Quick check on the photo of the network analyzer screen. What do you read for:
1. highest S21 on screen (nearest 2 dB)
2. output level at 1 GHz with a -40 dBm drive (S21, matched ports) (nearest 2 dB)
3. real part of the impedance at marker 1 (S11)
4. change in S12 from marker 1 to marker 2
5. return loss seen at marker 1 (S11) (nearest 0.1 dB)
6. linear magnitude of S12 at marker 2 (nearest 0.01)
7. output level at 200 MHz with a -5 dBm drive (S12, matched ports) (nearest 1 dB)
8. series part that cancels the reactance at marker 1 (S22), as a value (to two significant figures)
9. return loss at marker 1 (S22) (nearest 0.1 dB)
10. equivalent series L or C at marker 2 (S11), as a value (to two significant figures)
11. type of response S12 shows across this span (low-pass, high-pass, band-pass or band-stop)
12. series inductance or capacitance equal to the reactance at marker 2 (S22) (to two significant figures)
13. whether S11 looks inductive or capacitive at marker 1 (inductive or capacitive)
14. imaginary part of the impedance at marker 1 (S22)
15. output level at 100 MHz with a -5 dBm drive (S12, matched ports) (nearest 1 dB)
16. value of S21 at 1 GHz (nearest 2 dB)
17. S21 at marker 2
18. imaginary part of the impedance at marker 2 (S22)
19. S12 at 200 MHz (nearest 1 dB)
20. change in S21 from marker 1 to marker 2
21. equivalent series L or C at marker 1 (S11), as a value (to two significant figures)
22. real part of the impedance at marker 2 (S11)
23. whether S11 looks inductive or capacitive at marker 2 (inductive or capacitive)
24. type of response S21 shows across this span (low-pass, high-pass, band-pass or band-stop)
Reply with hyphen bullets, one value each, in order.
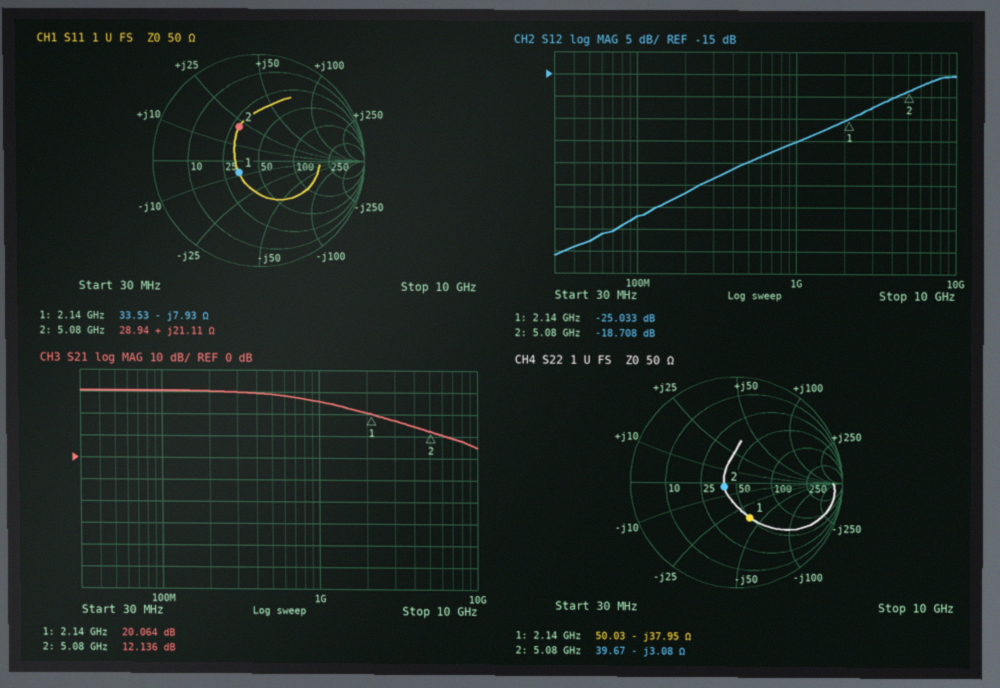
- 30 dB
- -14 dBm
- 33.53 Ω
- 6.325 dB
- 13.2 dB
- 0.12
- -47 dBm
- 2.8 nH
- 9.0 dB
- 660 pH
- high-pass
- 10 pF
- capacitive
- -37.95 Ω
- -52 dBm
- 26 dB
- 12.136 dB
- -3.08 Ω
- -42 dB
- -7.928 dB
- 9.4 pF
- 28.94 Ω
- inductive
- low-pass
